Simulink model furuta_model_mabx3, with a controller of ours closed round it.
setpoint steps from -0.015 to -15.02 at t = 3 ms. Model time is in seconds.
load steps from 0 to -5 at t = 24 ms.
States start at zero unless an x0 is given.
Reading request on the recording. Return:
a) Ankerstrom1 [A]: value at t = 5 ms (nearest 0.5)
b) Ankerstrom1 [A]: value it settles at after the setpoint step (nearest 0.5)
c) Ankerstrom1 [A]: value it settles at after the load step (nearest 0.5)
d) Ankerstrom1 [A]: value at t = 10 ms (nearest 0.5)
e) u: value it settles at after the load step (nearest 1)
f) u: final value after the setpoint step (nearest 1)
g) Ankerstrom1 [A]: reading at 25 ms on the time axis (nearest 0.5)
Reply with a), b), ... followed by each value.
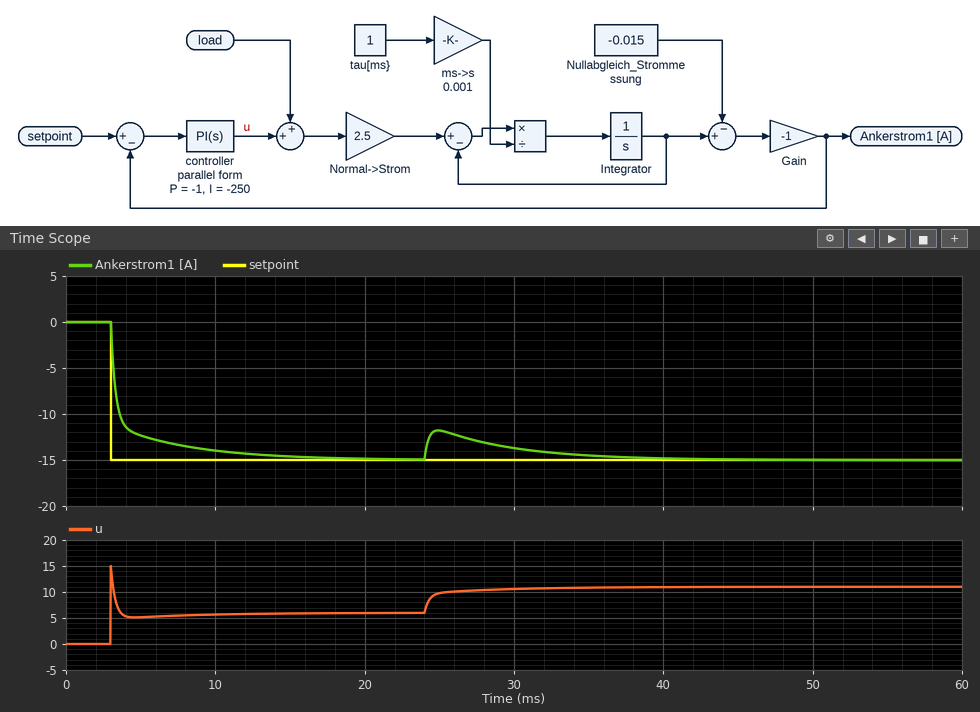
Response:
a) -12.5
b) -15.0
c) -15.0
d) -14.0
e) 11
f) 6
g) -12.0
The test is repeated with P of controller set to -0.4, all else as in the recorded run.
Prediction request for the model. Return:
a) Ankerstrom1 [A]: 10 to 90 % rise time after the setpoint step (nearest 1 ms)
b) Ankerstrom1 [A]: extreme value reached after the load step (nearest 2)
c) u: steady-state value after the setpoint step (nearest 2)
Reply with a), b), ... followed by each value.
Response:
a) 4 ms
b) -10
c) 6
